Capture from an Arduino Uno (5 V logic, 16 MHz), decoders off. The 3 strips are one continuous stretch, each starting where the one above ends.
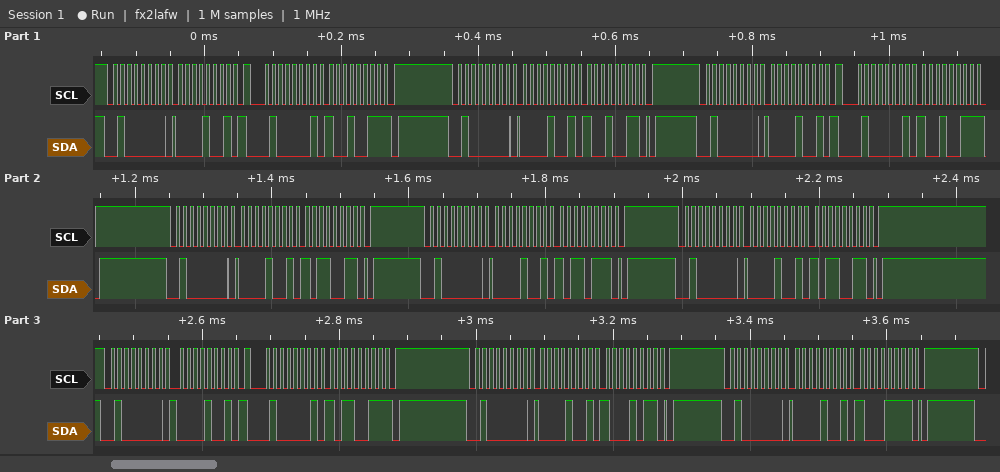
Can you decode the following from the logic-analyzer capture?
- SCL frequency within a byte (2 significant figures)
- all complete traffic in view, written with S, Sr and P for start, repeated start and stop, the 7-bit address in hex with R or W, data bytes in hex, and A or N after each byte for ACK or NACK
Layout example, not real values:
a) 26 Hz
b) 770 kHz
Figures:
a) 100 kHz
b) S 20W A 09 A Sr 20R A 93 N P S 20W A 09 A 93 A P S 20W A 09 A Sr 20R A 93 N P S 20W A 09 A B3 A P S 20W A 09 A B7 A P S 20W A 09 A B3 A P S 20W A 09 A Sr 20R A B3 N P S 20W A 09 A 8B A P S 20W A 09 A 8F A P
